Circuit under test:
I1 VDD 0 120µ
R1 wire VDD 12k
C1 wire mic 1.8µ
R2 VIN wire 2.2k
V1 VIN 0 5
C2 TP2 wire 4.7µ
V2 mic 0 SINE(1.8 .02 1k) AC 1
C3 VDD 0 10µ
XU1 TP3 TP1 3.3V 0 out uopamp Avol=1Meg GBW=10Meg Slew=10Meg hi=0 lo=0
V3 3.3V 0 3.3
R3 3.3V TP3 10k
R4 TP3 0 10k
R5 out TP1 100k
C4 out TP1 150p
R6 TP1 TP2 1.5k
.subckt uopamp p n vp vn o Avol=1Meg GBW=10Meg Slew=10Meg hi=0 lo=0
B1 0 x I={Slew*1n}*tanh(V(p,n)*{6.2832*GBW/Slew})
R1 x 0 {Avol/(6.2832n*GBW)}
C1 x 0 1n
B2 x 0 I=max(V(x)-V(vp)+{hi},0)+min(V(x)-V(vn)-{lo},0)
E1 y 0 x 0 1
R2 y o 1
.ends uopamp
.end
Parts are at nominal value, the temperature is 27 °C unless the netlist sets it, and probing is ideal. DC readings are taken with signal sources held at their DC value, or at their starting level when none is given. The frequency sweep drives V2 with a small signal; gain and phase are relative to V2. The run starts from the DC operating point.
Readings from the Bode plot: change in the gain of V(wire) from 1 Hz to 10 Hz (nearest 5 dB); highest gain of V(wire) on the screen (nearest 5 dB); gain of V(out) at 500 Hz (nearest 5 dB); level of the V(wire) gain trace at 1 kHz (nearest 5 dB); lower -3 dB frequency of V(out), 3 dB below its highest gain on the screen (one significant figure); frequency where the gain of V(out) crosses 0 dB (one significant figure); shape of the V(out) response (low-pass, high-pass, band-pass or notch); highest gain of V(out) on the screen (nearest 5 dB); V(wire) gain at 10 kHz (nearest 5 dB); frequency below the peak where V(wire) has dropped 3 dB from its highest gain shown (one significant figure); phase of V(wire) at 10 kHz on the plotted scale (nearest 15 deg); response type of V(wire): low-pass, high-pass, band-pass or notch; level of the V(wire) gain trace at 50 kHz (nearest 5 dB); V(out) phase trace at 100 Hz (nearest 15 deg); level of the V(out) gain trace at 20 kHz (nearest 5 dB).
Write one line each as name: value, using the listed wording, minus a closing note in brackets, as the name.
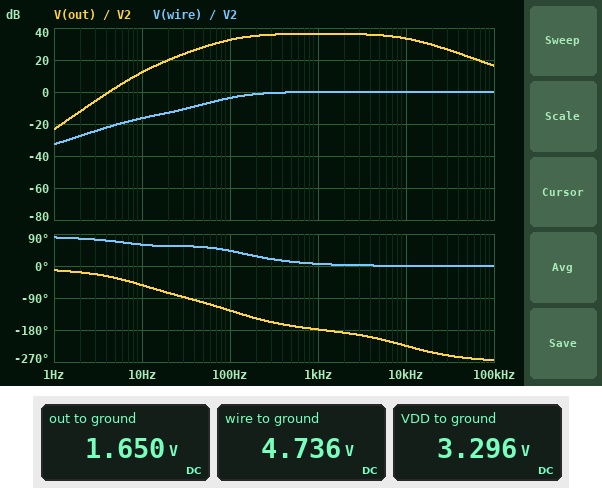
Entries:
change in the gain of V(wire) from 1 Hz to 10 Hz: 15 dB
highest gain of V(wire) on the screen: 0 dB
gain of V(out) at 500 Hz: 35 dB
level of the V(wire) gain trace at 1 kHz: 0 dB
lower -3 dB frequency of V(out), 3 dB below its highest gain on the screen: 100 Hz
frequency where the gain of V(out) crosses 0 dB: 4 Hz
shape of the V(out) response: band-pass
highest gain of V(out) on the screen: 35 dB
V(wire) gain at 10 kHz: 0 dB
frequency below the peak where V(wire) has dropped 3 dB from its highest gain shown: 100 Hz
phase of V(wire) at 10 kHz on the plotted scale: 0 deg
response type of V(wire): low-pass, high-pass, band-pass or notch: high-pass
level of the V(wire) gain trace at 50 kHz: 0 dB
V(out) phase trace at 100 Hz: -120 deg
level of the V(out) gain trace at 20 kHz: 30 dB
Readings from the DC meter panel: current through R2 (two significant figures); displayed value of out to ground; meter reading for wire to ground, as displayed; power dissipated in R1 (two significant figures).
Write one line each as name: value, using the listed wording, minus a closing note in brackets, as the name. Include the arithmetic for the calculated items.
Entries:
current through R2: (5 V - 4.736 V) / 2.2 kΩ = 120 µA
displayed value of out to ground: 1.650 V
meter reading for wire to ground, as displayed: 4.736 V
power dissipated in R1: (4.736 V - 3.296 V)^2 / 12 kΩ = 170 µW
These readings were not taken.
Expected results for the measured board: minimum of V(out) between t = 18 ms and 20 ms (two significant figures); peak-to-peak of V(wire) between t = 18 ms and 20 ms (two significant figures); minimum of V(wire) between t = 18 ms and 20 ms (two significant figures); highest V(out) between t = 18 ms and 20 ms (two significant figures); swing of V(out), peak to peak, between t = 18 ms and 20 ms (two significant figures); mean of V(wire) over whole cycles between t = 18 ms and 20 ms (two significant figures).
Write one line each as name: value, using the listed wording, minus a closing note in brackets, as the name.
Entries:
minimum of V(out) between t = 18 ms and 20 ms: 330 mV
peak-to-peak of V(wire) between t = 18 ms and 20 ms: 40 mV
minimum of V(wire) between t = 18 ms and 20 ms: 4.7 V
highest V(out) between t = 18 ms and 20 ms: 3.0 V
swing of V(out), peak to peak, between t = 18 ms and 20 ms: 2.6 V
mean of V(wire) over whole cycles between t = 18 ms and 20 ms: 4.7 V
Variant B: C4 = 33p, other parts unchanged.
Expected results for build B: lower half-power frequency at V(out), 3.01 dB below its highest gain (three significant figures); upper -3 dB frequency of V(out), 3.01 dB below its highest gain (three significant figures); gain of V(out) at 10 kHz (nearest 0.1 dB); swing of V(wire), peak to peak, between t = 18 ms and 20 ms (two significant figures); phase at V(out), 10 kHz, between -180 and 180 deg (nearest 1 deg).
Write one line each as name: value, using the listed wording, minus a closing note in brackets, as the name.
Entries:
lower half-power frequency at V(out), 3.01 dB below its highest gain: 120 Hz
upper -3 dB frequency of V(out), 3.01 dB below its highest gain: 36.7 kHz
gain of V(out) at 10 kHz: 36.2 dB
swing of V(wire), peak to peak, between t = 18 ms and 20 ms: 40 mV
phase at V(out), 10 kHz, between -180 and 180 deg: 165 deg
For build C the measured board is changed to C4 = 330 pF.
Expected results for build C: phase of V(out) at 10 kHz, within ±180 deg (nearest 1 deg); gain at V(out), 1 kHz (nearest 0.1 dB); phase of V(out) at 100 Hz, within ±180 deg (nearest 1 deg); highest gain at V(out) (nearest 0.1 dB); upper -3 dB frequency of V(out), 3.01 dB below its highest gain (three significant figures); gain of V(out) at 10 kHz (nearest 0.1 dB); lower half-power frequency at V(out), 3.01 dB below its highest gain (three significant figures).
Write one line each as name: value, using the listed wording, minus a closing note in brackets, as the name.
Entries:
phase of V(out) at 10 kHz, within ±180 deg: 116 deg
gain at V(out), 1 kHz: 36.2 dB
phase of V(out) at 100 Hz, within ±180 deg: -126 deg
highest gain at V(out): 36.3 dB
upper -3 dB frequency of V(out), 3.01 dB below its highest gain: 4.91 kHz
gain of V(out) at 10 kHz: 29.0 dB
lower half-power frequency at V(out), 3.01 dB below its highest gain: 115 Hz
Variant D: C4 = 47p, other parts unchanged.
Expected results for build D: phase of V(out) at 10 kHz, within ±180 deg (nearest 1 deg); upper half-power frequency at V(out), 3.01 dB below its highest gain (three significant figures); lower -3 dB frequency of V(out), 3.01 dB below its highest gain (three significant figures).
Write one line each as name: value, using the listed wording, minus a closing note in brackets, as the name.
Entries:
phase of V(out) at 10 kHz, within ±180 deg: 161 deg
upper half-power frequency at V(out), 3.01 dB below its highest gain: 27.8 kHz
lower -3 dB frequency of V(out), 3.01 dB below its highest gain: 120 Hz
